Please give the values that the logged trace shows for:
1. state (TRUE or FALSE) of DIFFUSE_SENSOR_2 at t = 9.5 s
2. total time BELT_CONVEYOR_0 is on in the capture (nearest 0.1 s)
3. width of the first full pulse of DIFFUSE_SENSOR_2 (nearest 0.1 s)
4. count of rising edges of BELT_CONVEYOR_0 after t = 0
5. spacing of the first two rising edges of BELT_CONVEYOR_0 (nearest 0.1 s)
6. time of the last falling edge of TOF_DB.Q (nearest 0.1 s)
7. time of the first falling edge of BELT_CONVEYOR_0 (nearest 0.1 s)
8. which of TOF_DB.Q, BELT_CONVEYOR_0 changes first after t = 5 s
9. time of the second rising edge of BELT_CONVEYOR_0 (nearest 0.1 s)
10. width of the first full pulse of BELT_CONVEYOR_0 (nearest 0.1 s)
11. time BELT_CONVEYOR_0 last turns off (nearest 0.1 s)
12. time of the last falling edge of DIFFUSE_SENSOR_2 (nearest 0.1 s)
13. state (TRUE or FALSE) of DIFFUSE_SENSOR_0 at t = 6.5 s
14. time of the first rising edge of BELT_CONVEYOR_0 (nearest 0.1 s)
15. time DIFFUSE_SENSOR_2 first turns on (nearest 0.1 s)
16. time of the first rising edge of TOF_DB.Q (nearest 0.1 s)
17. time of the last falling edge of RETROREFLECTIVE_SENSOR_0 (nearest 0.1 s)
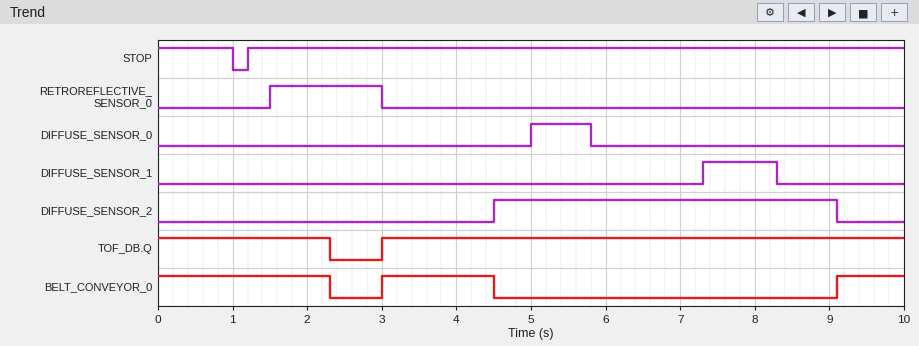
FALSE
4.7 s
4.6 s
2
6.1 s
2.3 s
2.3 s
BELT_CONVEYOR_0
9.1 s
1.5 s
4.5 s
9.1 s
FALSE
3.0 s
4.5 s
3.0 s
3.0 s
